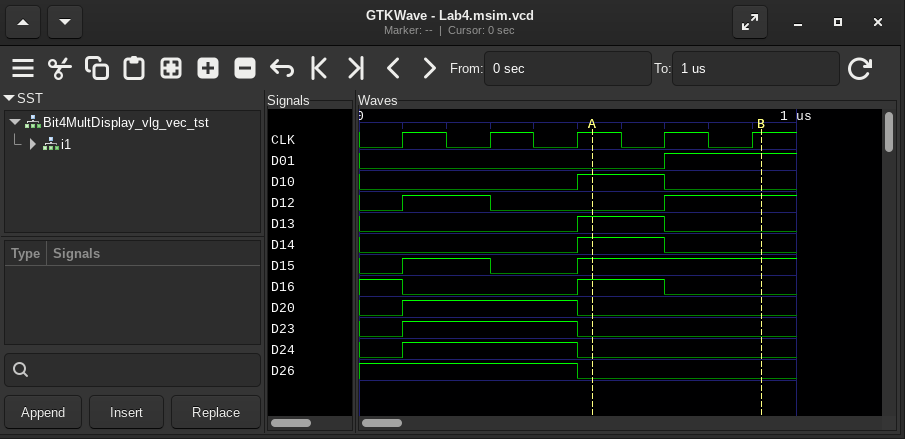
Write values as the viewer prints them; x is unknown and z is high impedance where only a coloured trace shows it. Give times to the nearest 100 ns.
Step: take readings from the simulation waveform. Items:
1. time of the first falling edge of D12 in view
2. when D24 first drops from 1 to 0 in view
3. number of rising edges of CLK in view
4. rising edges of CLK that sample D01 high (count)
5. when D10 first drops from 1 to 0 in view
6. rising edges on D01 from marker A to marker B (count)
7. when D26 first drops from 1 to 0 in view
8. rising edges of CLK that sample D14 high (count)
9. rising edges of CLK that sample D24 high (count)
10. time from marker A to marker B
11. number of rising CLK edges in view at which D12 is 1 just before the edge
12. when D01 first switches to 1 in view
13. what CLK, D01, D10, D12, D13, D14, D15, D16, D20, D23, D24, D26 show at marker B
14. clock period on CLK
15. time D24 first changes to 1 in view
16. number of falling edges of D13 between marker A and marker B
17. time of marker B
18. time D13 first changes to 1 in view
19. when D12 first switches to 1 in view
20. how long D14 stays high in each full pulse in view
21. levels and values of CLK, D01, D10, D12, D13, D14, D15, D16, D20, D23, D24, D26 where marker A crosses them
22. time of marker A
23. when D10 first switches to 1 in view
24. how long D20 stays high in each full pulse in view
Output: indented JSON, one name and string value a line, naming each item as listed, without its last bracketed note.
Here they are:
{
  "time of the first falling edge of D12 in view": "300 ns",
  "when D24 first drops from 1 to 0 in view": "500 ns",
  "number of rising edges of CLK in view": "5",
  "rising edges of CLK that sample D01 high": "1",
  "when D10 first drops from 1 to 0 in view": "700 ns",
  "rising edges on D01 from marker A to marker B": "1",
  "when D26 first drops from 1 to 0 in view": "500 ns",
  "rising edges of CLK that sample D14 high": "1",
  "rising edges of CLK that sample D24 high": "2",
  "time from marker A to marker B": "400 ns",
  "number of rising CLK edges in view at which D12 is 1 just before the edge": "2",
  "when D01 first switches to 1 in view": "700 ns",
  "what CLK, D01, D10, D12, D13, D14, D15, D16, D20, D23, D24, D26 show at marker B": "CLK=1, D01=1, D10=0, D12=1, D13=0, D14=0, D15=1, D16=0, D20=0, D23=0, D24=0, D26=0",
  "clock period on CLK": "200 ns",
  "time D24 first changes to 1 in view": "100 ns",
  "number of falling edges of D13 between marker A and marker B": "1",
  "time of marker B": "900 ns",
  "time D13 first changes to 1 in view": "500 ns",
  "when D12 first switches to 1 in view": "100 ns",
  "how long D14 stays high in each full pulse in view": "200 ns",
  "levels and values of CLK, D01, D10, D12, D13, D14, D15, D16, D20, D23, D24, D26 where marker A crosses them": "CLK=1, D01=0, D10=1, D12=0, D13=1, D14=1, D15=1, D16=1, D20=0, D23=0, D24=0, D26=0",
  "time of marker A": "500 ns",
  "when D10 first switches to 1 in view": "500 ns",
  "how long D20 stays high in each full pulse in view": "400 ns"
}
